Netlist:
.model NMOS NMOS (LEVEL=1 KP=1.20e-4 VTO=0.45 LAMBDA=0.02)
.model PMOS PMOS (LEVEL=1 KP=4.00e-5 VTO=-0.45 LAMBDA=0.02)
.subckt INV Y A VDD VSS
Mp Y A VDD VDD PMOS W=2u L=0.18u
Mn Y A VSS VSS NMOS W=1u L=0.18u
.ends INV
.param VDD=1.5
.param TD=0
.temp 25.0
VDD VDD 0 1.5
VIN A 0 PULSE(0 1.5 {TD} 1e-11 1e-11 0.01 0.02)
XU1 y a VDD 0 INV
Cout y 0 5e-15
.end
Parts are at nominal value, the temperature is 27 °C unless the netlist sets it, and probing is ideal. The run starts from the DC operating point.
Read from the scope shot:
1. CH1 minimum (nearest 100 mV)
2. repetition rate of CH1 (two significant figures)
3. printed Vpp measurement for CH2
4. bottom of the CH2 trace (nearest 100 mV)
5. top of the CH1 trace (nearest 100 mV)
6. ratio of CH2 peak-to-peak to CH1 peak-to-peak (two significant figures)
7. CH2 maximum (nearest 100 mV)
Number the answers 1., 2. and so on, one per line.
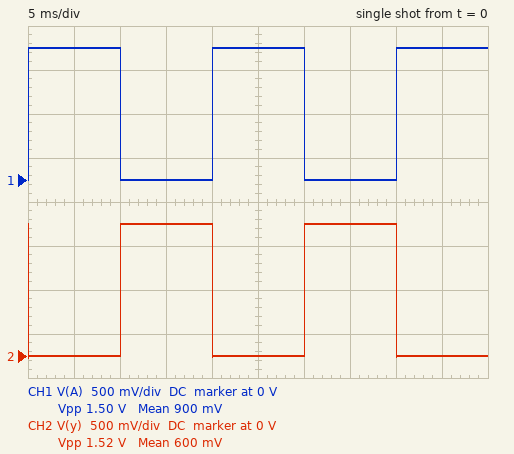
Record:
1. 0 V
2. 50 Hz
3. 1.52 V
4. 0 V
5. 1.5 V
6. 1.0
7. 1.5 V
